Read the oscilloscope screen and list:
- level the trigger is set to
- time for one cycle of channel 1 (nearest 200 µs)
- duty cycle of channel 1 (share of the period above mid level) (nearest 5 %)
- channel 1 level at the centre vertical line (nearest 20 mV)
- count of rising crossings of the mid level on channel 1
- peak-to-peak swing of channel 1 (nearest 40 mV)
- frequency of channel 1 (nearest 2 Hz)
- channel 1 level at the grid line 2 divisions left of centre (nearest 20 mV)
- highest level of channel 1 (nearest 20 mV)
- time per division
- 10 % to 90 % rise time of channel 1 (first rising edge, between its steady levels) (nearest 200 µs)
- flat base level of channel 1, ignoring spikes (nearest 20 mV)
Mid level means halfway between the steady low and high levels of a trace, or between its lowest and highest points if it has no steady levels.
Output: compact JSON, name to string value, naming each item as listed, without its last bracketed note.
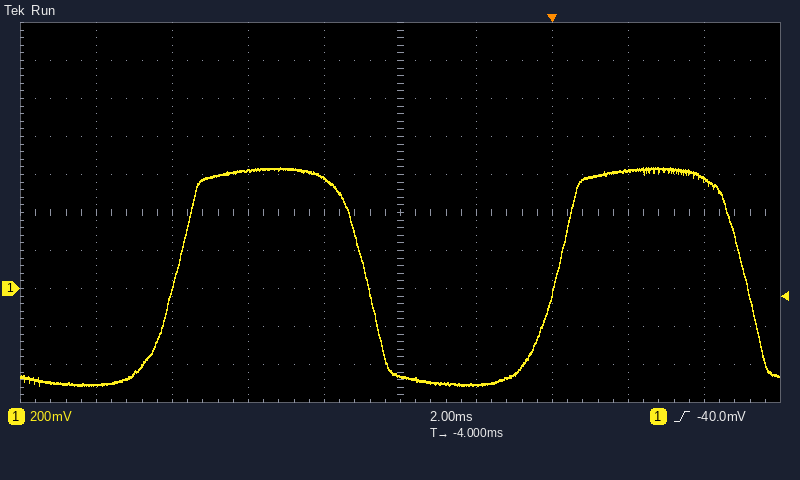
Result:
{"level the trigger is set to": "-40.0 mV", "time for one cycle of channel 1": "10.0 ms", "duty cycle of channel 1 (share of the period above mid level)": "50 %", "channel 1 level at the centre vertical line": "-460 mV", "count of rising crossings of the mid level on channel 1": "2", "peak-to-peak swing of channel 1": "1.16 V", "frequency of channel 1": "100 Hz", "channel 1 level at the grid line 2 divisions left of centre": "620 mV", "highest level of channel 1": "640 mV", "time per division": "2 ms", "10 % to 90 % rise time of channel 1 (first rising edge, between its steady levels)": "1.4 ms", "flat base level of channel 1, ignoring spikes": "-500 mV"}
